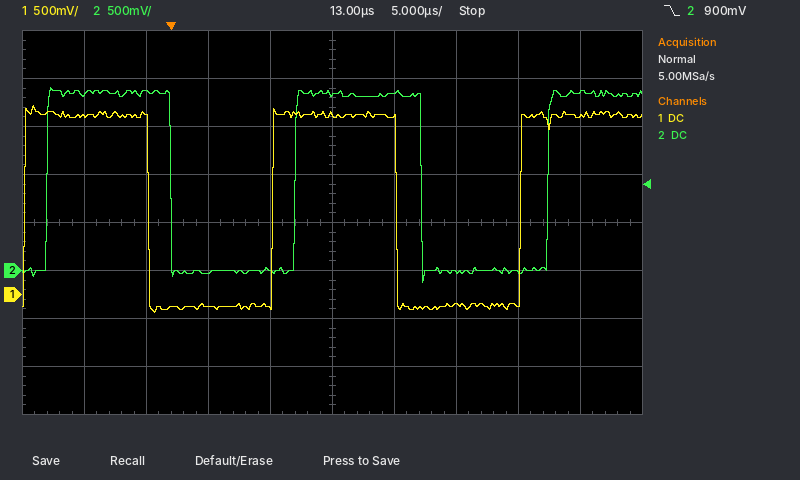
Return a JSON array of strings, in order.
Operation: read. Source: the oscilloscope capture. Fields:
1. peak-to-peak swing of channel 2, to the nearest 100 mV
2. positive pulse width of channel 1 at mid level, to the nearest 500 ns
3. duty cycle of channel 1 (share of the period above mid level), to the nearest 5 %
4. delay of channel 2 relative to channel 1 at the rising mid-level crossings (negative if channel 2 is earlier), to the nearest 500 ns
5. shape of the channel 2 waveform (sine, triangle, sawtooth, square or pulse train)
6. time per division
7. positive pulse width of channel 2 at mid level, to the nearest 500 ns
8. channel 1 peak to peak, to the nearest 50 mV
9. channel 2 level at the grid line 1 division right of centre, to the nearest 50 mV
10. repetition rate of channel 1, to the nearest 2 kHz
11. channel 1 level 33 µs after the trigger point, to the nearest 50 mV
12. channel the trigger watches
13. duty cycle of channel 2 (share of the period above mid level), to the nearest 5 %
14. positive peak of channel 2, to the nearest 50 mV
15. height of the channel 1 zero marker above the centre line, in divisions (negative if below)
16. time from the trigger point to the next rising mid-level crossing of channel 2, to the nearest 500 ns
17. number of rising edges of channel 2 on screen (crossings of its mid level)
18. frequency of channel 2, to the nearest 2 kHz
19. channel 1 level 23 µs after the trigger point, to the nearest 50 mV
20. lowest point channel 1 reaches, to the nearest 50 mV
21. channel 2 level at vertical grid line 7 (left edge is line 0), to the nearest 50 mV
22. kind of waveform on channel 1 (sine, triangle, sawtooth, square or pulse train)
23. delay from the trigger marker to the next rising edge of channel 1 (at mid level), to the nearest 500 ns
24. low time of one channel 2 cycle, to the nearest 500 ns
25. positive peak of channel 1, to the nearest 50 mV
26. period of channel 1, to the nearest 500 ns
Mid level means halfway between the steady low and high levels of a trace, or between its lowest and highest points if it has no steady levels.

["2.00 V", "10.0 µs", "50 %", "+2.0 µs", "square", "5 µs", "10.0 µs", "2.15 V", "1.85 V", "50 kHz", "1.85 V", "channel 2", "50 %", "1.90 V", "-1.5 div", "10.0 µs", "3", "50 kHz", "-100 mV", "-200 mV", "0 mV", "square", "8.0 µs", "10.0 µs", "1.95 V", "20.0 µs"]
